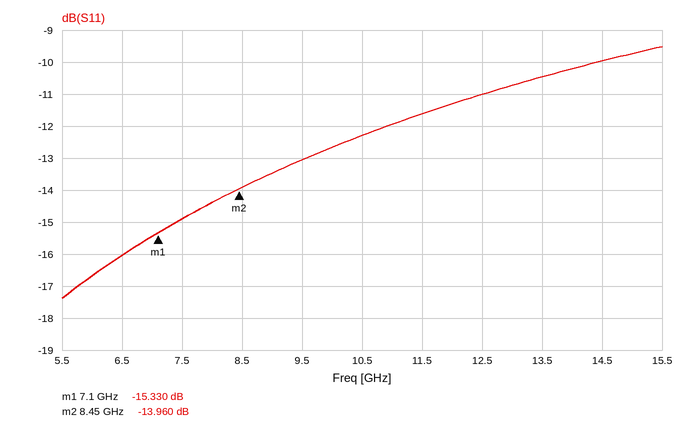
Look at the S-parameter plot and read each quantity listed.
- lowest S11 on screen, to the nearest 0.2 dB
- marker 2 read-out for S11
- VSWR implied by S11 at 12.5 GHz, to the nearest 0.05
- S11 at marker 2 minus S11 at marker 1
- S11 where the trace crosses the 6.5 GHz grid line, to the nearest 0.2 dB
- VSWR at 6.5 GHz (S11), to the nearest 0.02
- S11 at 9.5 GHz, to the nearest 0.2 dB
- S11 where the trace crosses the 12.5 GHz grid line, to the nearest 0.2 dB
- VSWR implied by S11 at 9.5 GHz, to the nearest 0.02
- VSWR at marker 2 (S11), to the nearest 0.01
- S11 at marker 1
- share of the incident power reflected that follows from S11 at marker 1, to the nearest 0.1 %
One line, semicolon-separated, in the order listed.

-17.4 dB; -13.960 dB; 1.80; 1.370 dB; -16.0 dB; 1.38; -13.0 dB; -11.0 dB; 1.58; 1.50; -15.330 dB; 2.9 %
